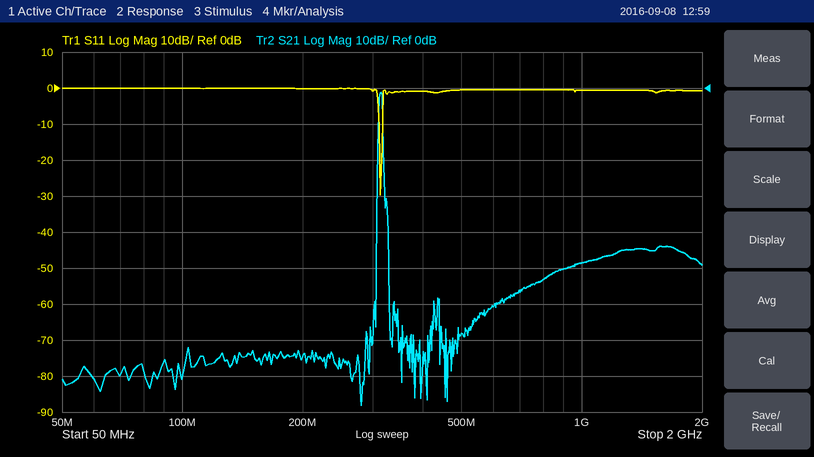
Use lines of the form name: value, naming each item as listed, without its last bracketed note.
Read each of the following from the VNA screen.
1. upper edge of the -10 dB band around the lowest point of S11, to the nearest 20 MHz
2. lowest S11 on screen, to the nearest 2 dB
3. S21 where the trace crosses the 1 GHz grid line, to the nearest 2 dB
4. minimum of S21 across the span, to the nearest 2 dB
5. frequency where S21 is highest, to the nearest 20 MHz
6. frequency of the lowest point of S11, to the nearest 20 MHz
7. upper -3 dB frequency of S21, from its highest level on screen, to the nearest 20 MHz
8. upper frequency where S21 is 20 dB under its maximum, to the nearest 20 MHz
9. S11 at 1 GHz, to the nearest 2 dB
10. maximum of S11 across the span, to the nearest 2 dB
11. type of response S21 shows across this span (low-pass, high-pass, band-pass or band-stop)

upper edge of the -10 dB band around the lowest point of S11, to the nearest 20 MHz: 320 MHz
lowest S11 on screen, to the nearest 2 dB: -30 dB
S21 where the trace crosses the 1 GHz grid line, to the nearest 2 dB: -48 dB
minimum of S21 across the span, to the nearest 2 dB: -88 dB
frequency where S21 is highest, to the nearest 20 MHz: 320 MHz
frequency of the lowest point of S11, to the nearest 20 MHz: 320 MHz
upper -3 dB frequency of S21, from its highest level on screen, to the nearest 20 MHz: 320 MHz
upper frequency where S21 is 20 dB under its maximum, to the nearest 20 MHz: 320 MHz
S11 at 1 GHz, to the nearest 2 dB: 0 dB
maximum of S11 across the span, to the nearest 2 dB: 0 dB
type of response S21 shows across this span: band-pass
